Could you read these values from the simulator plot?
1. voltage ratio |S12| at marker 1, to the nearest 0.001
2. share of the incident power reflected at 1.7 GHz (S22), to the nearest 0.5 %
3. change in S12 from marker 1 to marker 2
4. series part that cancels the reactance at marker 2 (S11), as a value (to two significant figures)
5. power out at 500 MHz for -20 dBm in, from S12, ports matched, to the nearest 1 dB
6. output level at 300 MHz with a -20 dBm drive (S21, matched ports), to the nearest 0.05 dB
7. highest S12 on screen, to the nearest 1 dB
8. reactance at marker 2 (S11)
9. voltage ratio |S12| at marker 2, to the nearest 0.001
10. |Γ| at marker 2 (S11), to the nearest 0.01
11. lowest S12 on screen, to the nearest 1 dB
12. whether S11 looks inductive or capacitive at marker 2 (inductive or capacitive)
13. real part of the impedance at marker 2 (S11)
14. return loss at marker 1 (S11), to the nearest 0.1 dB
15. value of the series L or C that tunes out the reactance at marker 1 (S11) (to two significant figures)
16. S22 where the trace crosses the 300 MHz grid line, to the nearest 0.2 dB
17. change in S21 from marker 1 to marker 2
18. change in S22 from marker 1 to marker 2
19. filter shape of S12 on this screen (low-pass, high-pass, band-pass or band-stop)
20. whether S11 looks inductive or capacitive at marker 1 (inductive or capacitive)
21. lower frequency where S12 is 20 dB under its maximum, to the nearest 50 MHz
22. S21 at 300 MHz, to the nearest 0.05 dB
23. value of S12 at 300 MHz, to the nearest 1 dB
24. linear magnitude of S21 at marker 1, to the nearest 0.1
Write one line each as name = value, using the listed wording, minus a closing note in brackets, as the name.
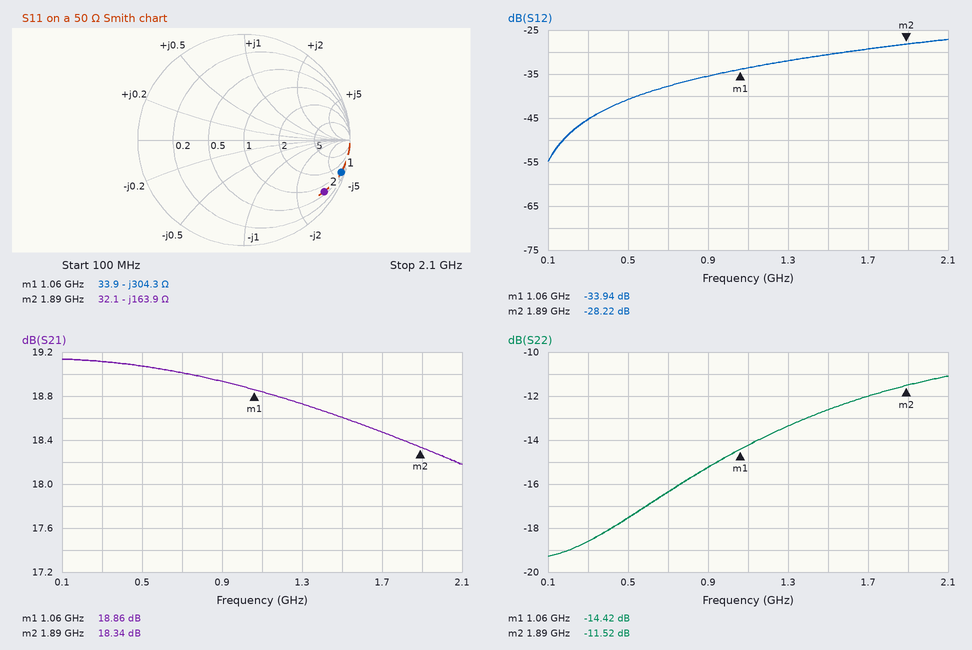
voltage ratio |S12| at marker 1, to the nearest 0.001 = 0.020
share of the incident power reflected at 1.7 GHz (S22), to the nearest 0.5 % = 6.5 %
change in S12 from marker 1 to marker 2 = 5.72 dB
series part that cancels the reactance at marker 2 (S11), as a value = 14 nH
power out at 500 MHz for -20 dBm in, from S12, ports matched, to the nearest 1 dB = -61 dBm
output level at 300 MHz with a -20 dBm drive (S21, matched ports), to the nearest 0.05 dB = -0.90 dBm
highest S12 on screen, to the nearest 1 dB = -27 dB
reactance at marker 2 = -163.9 Ω
voltage ratio |S12| at marker 2, to the nearest 0.001 = 0.039
|Γ| at marker 2 (S11), to the nearest 0.01 = 0.90
lowest S12 on screen, to the nearest 1 dB = -55 dB
whether S11 looks inductive or capacitive at marker 2 = capacitive
real part of the impedance at marker 2 = 32.1 Ω
return loss at marker 1 (S11), to the nearest 0.1 dB = 0.3 dB
value of the series L or C that tunes out the reactance at marker 1 (S11) = 46 nH
S22 where the trace crosses the 300 MHz grid line, to the nearest 0.2 dB = -18.6 dB
change in S21 from marker 1 to marker 2 = -0.52 dB
change in S22 from marker 1 to marker 2 = 2.90 dB
filter shape of S12 on this screen = high-pass
whether S11 looks inductive or capacitive at marker 1 = capacitive
lower frequency where S12 is 20 dB under its maximum, to the nearest 50 MHz = 250 MHz
S21 at 300 MHz, to the nearest 0.05 dB = 19.10 dB
value of S12 at 300 MHz, to the nearest 1 dB = -45 dB
linear magnitude of S21 at marker 1, to the nearest 0.1 = 8.8
